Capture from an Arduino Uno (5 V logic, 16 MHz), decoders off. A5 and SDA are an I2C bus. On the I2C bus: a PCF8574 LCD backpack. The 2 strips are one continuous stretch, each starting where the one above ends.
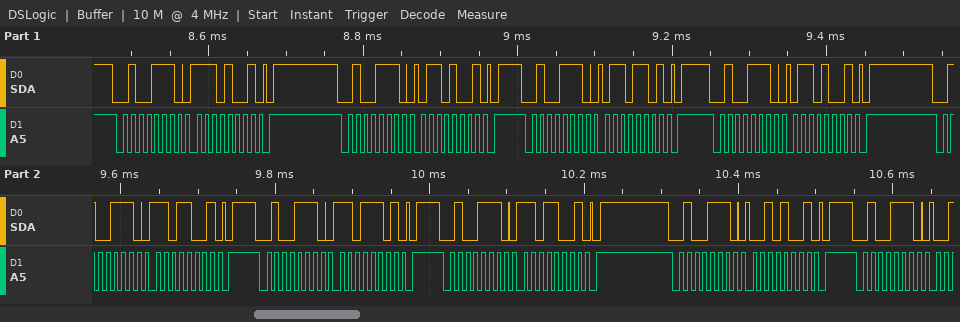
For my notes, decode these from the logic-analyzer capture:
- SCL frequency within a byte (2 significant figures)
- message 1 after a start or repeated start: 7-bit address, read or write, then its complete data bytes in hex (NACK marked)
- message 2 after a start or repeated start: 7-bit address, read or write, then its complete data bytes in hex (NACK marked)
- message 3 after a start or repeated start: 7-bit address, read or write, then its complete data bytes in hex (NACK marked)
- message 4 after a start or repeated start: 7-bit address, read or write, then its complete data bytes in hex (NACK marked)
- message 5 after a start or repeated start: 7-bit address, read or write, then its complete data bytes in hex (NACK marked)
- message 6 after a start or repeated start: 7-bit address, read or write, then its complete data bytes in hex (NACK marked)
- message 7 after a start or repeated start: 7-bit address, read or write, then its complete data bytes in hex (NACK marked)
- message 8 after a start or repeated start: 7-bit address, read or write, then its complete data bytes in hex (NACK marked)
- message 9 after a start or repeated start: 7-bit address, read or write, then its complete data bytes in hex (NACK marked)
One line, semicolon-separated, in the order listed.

100 kHz; 0x27 write: E9; 0x27 write: 69; 0x27 write: 6D; 0x27 write: 69; 0x27 write: D9; 0x27 write: DD; 0x27 write: D9; 0x27 write: 29; 0x27 write
